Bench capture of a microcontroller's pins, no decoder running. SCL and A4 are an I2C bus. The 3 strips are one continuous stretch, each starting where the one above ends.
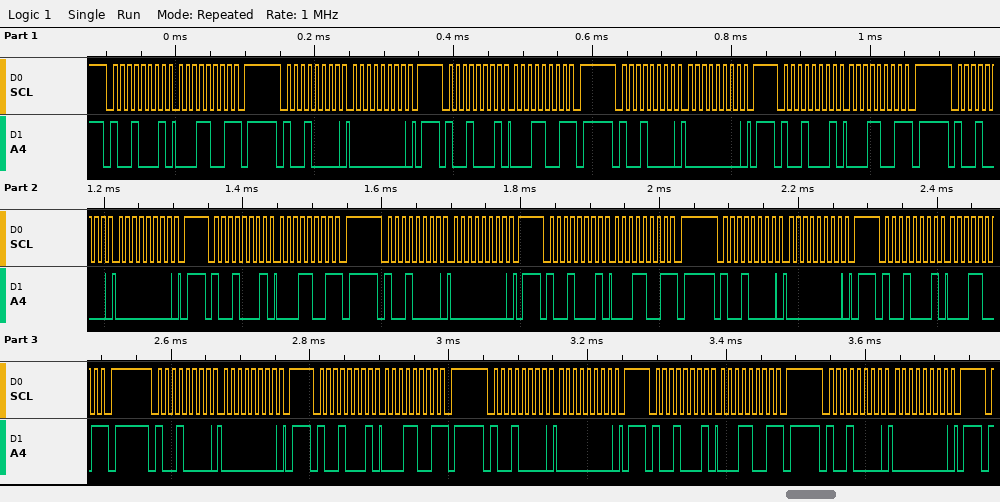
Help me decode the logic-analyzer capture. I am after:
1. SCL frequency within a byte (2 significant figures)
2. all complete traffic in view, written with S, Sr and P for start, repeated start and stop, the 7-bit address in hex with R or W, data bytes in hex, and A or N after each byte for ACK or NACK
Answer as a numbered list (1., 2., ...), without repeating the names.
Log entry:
1. 100 kHz
2. S 48R A 19 N P S 48W A 00 A P S 48R A 19 N P S 48W A 00 A P S 48R A 19 N P S 48W A 00 A P S 48R A 19 N P S 48W A 00 A P S 48R A 19 N P S 48W A 00 A P S 48R A 19 N P S 48W A 00 A P S 48R A 19 N P S 48W A 00 A P S 48R A 19 N P S 48W A 00 A P
